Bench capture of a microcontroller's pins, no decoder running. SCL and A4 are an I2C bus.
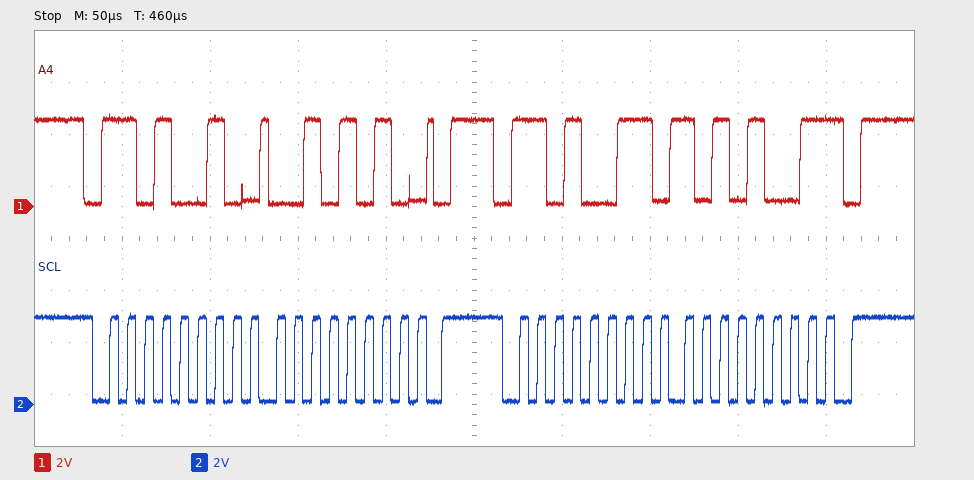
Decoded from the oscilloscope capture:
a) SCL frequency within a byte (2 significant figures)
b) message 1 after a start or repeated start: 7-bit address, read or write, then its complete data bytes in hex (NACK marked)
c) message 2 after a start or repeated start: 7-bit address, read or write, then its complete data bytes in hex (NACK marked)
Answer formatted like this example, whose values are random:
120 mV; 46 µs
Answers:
100 kHz; 0x69 write: 2A; 0x69 read: A9 NACK
